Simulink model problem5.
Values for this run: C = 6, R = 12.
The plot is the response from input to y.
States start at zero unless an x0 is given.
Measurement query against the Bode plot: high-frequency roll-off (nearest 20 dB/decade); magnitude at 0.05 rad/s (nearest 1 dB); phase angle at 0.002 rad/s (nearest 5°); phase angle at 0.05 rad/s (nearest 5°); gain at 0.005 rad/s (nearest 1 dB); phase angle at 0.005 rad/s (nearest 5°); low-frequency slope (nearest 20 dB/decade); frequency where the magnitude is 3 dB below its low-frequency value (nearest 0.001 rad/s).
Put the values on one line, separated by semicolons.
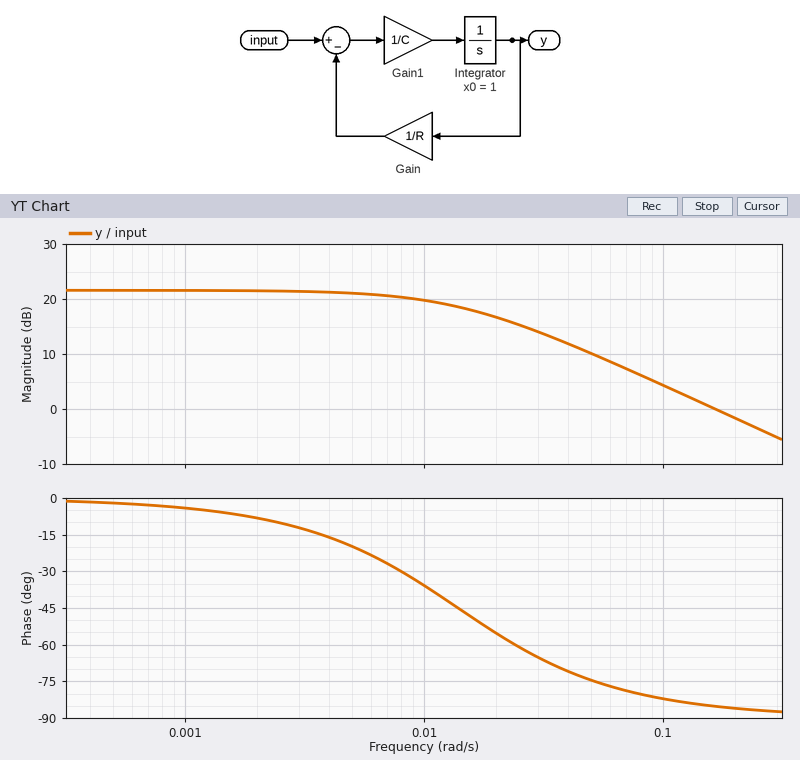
-20 dB/decade; 10 dB; -10°; -75°; 21 dB; -20°; 0 dB/decade; 0.014 rad/s
